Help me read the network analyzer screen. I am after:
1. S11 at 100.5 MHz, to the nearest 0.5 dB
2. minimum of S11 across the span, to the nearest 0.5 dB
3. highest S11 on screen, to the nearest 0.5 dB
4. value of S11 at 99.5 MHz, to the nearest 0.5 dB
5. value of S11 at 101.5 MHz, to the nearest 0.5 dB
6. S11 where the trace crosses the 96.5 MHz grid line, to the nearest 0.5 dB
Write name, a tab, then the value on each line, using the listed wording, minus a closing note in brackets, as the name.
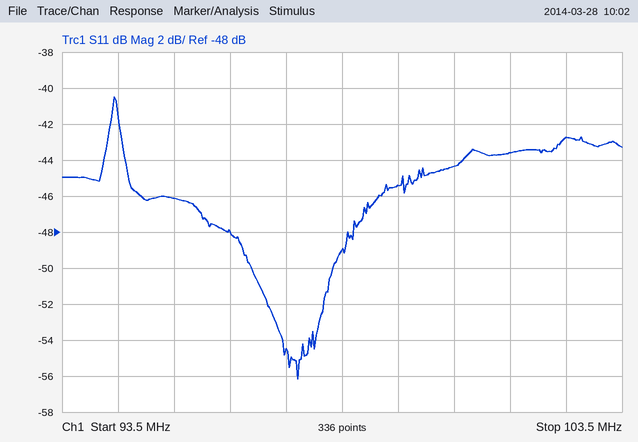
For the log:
S11 at 100.5 MHz, to the nearest 0.5 dB	-44.5 dB
minimum of S11 across the span, to the nearest 0.5 dB	-56.0 dB
highest S11 on screen, to the nearest 0.5 dB	-40.5 dB
value of S11 at 99.5 MHz, to the nearest 0.5 dB	-45.5 dB
value of S11 at 101.5 MHz, to the nearest 0.5 dB	-43.5 dB
S11 where the trace crosses the 96.5 MHz grid line, to the nearest 0.5 dB	-48.0 dB
